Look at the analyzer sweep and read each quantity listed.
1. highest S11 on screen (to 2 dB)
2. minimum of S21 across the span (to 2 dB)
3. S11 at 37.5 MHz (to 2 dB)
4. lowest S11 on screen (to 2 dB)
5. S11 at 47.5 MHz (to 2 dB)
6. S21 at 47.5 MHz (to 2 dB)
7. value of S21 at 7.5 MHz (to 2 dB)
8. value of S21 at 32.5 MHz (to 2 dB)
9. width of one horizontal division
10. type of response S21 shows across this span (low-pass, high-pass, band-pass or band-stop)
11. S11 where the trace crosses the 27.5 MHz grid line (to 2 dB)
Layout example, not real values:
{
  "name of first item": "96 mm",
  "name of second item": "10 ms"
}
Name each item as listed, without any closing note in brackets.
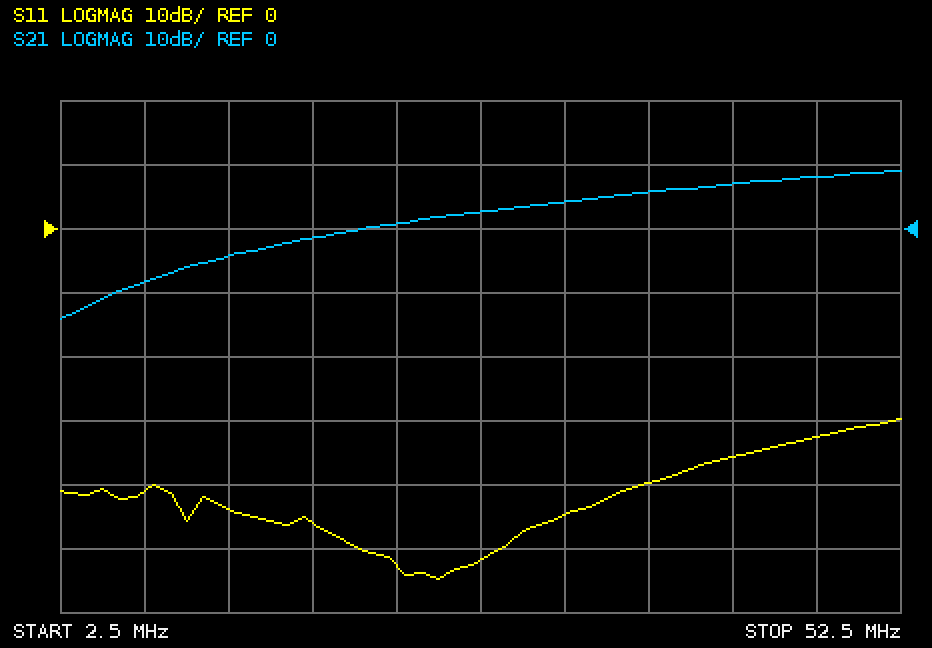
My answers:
{
  "highest S11 on screen": "-30 dB",
  "minimum of S21 across the span": "-14 dB",
  "S11 at 37.5 MHz": "-40 dB",
  "lowest S11 on screen": "-54 dB",
  "S11 at 47.5 MHz": "-32 dB",
  "S21 at 47.5 MHz": "8 dB",
  "value of S21 at 7.5 MHz": "-8 dB",
  "value of S21 at 32.5 MHz": "4 dB",
  "width of one horizontal division": "5 MHz",
  "type of response S21 shows across this span": "high-pass",
  "S11 where the trace crosses the 27.5 MHz grid line": "-52 dB"
}
